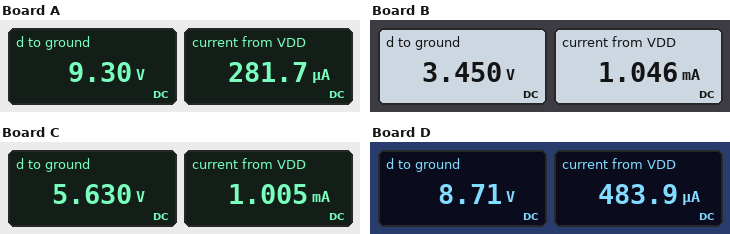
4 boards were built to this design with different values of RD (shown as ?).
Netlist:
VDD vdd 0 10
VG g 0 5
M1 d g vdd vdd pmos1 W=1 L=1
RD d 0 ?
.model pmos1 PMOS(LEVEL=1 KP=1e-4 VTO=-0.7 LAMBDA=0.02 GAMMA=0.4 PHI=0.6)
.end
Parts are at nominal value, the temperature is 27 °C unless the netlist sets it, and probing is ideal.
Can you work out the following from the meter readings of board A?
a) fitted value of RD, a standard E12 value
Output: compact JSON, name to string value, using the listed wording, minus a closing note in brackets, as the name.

{"fitted value of RD, a standard E12 value": "33 kΩ"}
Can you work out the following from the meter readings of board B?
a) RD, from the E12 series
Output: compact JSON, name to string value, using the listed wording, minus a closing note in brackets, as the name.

{"RD, from the E12 series": "3.3 kΩ"}
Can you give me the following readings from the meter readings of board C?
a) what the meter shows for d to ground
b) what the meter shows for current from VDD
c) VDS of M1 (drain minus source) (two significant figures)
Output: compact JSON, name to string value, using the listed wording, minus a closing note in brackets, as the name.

{"what the meter shows for d to ground": "5.630 V", "what the meter shows for current from VDD": "1.005 mA", "VDS of M1 (drain minus source)": "-4.4 V"}
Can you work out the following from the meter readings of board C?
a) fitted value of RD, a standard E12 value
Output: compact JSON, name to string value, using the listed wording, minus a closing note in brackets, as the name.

{"fitted value of RD, a standard E12 value": "5.6 kΩ"}
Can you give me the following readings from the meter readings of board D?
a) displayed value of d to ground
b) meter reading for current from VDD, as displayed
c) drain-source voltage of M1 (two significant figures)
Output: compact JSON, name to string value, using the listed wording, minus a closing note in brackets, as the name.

{"displayed value of d to ground": "8.71 V", "meter reading for current from VDD, as displayed": "483.9 µA", "drain-source voltage of M1": "-1.3 V"}
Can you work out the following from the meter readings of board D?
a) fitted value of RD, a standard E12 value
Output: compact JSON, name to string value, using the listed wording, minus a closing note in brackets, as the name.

{"fitted value of RD, a standard E12 value": "18 kΩ"}
